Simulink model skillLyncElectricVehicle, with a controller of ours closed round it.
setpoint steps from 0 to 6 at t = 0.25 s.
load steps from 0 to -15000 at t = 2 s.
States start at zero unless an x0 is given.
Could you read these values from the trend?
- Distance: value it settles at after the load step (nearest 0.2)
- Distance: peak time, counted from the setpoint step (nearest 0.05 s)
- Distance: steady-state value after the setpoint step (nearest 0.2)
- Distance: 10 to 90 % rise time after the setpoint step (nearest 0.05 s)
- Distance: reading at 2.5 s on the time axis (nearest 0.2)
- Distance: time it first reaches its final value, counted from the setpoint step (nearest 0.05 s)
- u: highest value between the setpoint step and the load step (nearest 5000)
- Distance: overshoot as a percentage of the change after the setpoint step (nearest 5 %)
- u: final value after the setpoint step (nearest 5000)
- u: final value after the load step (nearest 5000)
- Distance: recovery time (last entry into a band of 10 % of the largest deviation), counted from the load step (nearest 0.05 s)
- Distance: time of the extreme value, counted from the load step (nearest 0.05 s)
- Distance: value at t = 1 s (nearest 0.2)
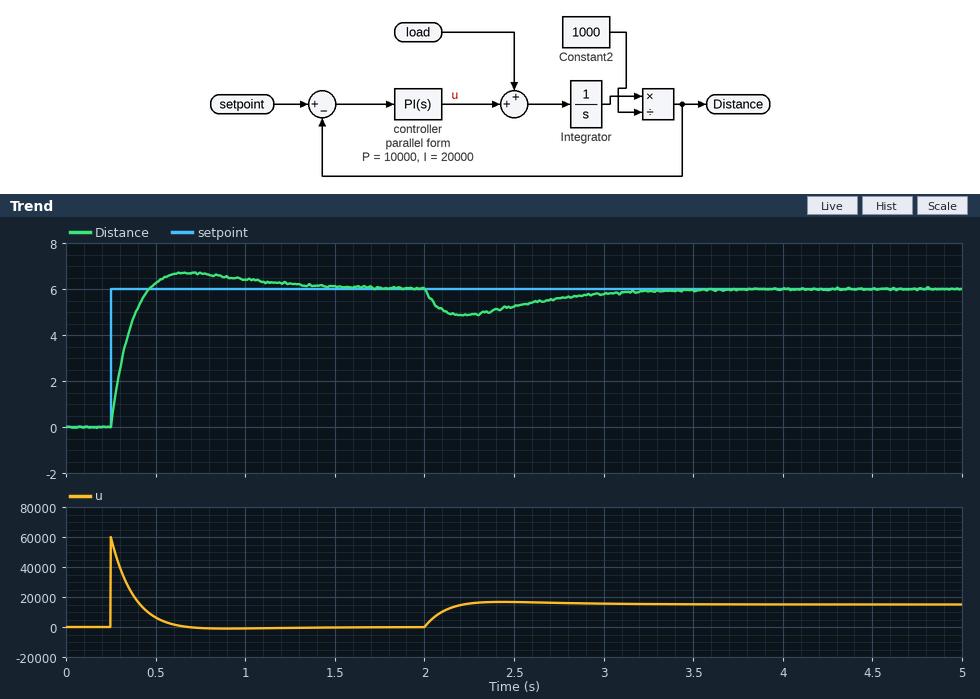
6.0
0.45 s
6.0
0.15 s
5.2
0.20 s
60000
10 %
0
15000
1.20 s
0.20 s
6.4
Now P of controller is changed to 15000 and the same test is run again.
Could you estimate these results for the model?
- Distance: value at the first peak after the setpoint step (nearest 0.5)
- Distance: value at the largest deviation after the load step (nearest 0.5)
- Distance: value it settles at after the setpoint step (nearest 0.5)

6.5
5.0
6.0
